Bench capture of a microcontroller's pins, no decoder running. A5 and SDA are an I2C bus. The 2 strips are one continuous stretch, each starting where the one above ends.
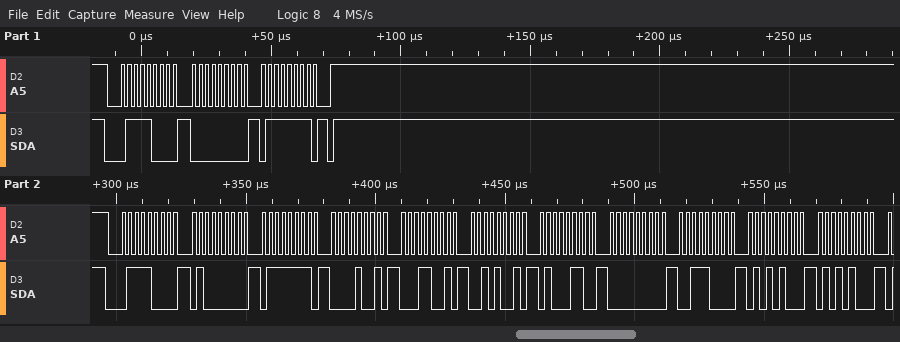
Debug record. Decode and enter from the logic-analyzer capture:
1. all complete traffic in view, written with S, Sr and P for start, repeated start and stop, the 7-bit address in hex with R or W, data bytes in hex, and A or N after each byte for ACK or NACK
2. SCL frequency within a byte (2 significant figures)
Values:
S 3CW A 00 A 7F A P S 3CW A 40 A 7F A 09 A 19 A 29 A 46 A 00 A 38 A 54 A 54 A
400 kHz
